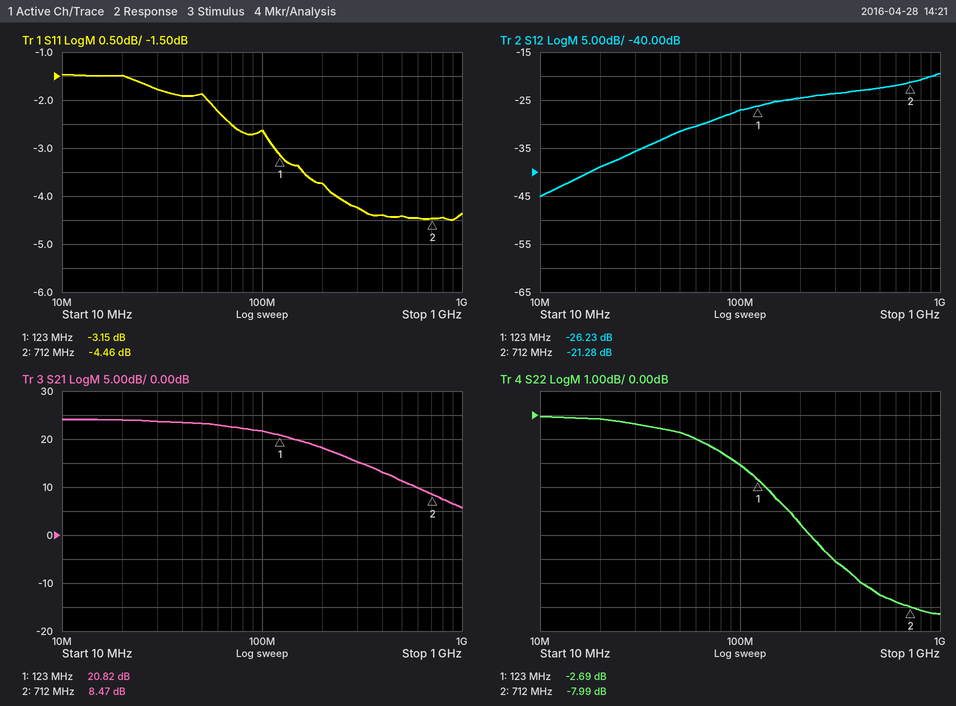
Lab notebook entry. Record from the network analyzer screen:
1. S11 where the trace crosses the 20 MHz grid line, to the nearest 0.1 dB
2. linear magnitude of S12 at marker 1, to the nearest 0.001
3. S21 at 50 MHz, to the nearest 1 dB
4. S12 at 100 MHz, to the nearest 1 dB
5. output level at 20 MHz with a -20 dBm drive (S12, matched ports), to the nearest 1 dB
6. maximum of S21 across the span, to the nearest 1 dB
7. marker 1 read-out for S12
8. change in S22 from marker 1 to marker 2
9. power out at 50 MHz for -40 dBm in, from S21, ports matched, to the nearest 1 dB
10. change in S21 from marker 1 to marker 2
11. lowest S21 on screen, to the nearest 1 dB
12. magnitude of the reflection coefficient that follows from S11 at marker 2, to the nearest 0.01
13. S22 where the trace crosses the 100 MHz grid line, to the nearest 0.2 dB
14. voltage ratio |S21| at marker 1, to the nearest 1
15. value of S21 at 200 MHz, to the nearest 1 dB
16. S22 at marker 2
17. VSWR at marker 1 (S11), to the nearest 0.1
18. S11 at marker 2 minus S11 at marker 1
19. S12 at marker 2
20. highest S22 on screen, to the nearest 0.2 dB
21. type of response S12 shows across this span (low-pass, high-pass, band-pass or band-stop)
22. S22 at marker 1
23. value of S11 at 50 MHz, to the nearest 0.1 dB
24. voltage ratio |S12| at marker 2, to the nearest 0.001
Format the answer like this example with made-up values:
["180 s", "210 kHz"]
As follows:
["-1.5 dB", "0.049", "23 dB", "-27 dB", "-59 dBm", "24 dB", "-26.23 dB", "-5.30 dB", "-17 dBm", "-12.35 dB", "6 dB", "0.60", "-2.0 dB", "11", "18 dB", "-7.99 dB", "5.6", "-1.31 dB", "-21.28 dB", "0.0 dB", "high-pass", "-2.69 dB", "-1.9 dB", "0.086"]
